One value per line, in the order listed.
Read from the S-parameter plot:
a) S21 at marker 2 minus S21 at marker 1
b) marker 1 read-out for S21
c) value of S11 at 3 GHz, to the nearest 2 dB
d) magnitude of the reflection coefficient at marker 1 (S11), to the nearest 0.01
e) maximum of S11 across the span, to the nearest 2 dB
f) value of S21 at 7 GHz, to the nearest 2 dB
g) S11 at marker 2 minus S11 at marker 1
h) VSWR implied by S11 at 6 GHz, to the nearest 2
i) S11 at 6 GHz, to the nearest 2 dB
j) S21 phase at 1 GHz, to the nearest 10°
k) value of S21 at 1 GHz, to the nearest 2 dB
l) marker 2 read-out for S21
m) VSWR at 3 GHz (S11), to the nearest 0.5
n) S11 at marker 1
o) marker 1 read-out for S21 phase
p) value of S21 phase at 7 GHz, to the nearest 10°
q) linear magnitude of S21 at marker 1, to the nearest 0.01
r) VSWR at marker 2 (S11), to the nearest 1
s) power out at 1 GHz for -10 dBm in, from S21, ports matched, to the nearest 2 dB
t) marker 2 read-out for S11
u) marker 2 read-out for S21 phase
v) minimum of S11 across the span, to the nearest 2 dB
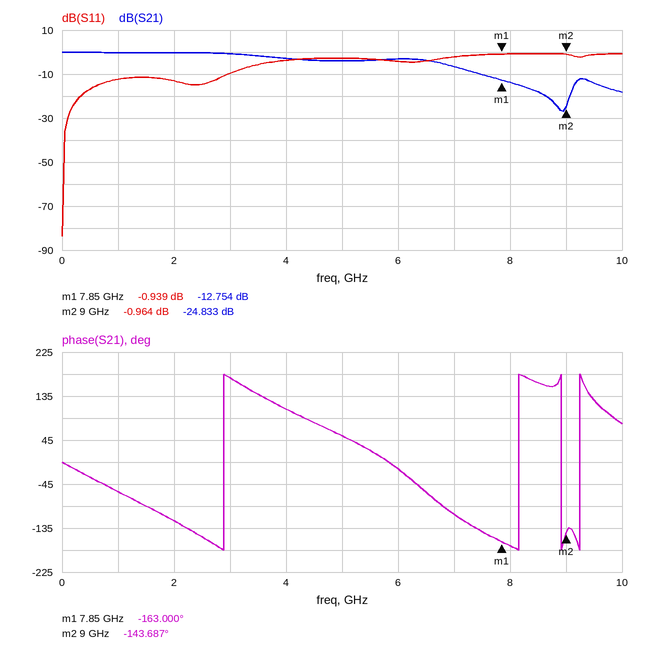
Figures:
-12.079 dB
-12.754 dB
-10 dB
0.90
0 dB
-6 dB
-0.025 dB
4
-4 dB
-60°
0 dB
-24.833 dB
2.0
-0.939 dB
-163.000°
-110°
0.23
18
-10 dBm
-0.964 dB
-143.687°
-84 dB
